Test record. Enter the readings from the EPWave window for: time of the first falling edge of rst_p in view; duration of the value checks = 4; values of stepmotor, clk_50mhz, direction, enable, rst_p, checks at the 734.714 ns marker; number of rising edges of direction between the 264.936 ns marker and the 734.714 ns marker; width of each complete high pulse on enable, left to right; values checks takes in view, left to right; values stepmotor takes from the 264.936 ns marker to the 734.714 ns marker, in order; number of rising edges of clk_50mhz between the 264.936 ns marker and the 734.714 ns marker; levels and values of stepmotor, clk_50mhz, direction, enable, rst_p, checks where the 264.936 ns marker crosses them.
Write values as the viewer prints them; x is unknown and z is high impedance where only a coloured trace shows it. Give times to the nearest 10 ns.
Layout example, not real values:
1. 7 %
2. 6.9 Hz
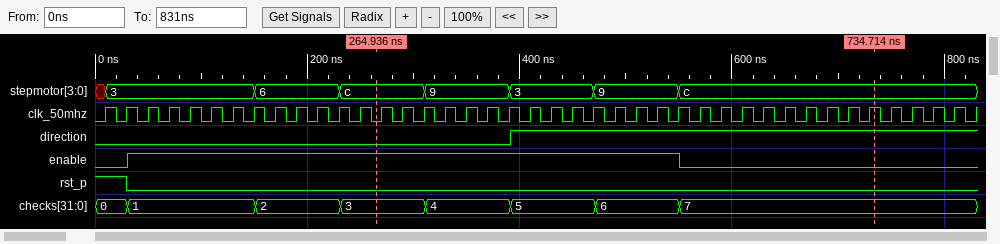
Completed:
1. 30 ns
2. 80 ns
3. stepmotor=c, clk_50mhz=1, direction=1, enable=0, rst_p=0, checks=7
4. 1
5. 520 ns
6. 0, 1, 2, 3, 4, 5, 6, 7
7. c, 9, 3, 9, c
8. 24
9. stepmotor=c, clk_50mhz=0, direction=0, enable=1, rst_p=0, checks=3
